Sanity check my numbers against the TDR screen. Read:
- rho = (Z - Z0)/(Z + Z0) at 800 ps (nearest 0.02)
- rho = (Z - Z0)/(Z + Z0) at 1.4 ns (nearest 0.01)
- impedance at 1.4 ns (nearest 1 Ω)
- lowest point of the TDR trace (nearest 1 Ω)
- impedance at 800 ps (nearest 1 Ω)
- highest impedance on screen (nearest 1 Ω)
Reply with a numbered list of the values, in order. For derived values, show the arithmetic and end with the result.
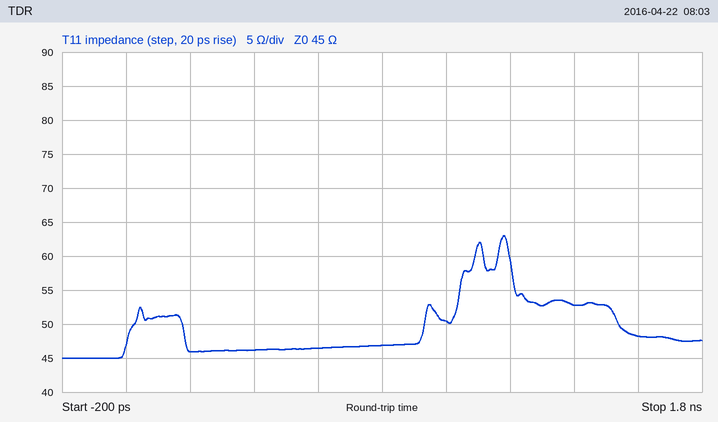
1. (47 − 45)/(47 + 45) ≈ +0.02
2. (53 − 45)/(53 + 45) ≈ +0.08
3. 53 Ω
4. 45 Ω
5. 47 Ω
6. 63 Ω
